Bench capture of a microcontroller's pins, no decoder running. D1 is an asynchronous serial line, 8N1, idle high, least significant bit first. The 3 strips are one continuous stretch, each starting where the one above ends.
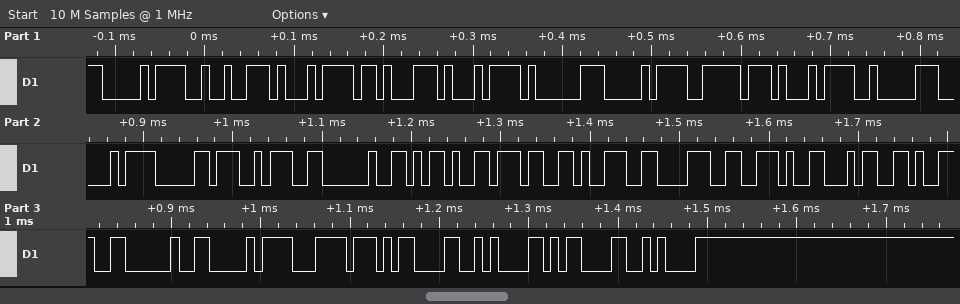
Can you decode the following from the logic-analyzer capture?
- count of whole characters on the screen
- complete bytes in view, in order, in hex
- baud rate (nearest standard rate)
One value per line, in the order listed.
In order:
28
D0 92 D1 8B D1 81 D0 BE D1 82 D0 B0 3A 20 2D 37 39 38 2E 34 39 20 D0 BC 0D 0A 0D 0A
115200 baud
